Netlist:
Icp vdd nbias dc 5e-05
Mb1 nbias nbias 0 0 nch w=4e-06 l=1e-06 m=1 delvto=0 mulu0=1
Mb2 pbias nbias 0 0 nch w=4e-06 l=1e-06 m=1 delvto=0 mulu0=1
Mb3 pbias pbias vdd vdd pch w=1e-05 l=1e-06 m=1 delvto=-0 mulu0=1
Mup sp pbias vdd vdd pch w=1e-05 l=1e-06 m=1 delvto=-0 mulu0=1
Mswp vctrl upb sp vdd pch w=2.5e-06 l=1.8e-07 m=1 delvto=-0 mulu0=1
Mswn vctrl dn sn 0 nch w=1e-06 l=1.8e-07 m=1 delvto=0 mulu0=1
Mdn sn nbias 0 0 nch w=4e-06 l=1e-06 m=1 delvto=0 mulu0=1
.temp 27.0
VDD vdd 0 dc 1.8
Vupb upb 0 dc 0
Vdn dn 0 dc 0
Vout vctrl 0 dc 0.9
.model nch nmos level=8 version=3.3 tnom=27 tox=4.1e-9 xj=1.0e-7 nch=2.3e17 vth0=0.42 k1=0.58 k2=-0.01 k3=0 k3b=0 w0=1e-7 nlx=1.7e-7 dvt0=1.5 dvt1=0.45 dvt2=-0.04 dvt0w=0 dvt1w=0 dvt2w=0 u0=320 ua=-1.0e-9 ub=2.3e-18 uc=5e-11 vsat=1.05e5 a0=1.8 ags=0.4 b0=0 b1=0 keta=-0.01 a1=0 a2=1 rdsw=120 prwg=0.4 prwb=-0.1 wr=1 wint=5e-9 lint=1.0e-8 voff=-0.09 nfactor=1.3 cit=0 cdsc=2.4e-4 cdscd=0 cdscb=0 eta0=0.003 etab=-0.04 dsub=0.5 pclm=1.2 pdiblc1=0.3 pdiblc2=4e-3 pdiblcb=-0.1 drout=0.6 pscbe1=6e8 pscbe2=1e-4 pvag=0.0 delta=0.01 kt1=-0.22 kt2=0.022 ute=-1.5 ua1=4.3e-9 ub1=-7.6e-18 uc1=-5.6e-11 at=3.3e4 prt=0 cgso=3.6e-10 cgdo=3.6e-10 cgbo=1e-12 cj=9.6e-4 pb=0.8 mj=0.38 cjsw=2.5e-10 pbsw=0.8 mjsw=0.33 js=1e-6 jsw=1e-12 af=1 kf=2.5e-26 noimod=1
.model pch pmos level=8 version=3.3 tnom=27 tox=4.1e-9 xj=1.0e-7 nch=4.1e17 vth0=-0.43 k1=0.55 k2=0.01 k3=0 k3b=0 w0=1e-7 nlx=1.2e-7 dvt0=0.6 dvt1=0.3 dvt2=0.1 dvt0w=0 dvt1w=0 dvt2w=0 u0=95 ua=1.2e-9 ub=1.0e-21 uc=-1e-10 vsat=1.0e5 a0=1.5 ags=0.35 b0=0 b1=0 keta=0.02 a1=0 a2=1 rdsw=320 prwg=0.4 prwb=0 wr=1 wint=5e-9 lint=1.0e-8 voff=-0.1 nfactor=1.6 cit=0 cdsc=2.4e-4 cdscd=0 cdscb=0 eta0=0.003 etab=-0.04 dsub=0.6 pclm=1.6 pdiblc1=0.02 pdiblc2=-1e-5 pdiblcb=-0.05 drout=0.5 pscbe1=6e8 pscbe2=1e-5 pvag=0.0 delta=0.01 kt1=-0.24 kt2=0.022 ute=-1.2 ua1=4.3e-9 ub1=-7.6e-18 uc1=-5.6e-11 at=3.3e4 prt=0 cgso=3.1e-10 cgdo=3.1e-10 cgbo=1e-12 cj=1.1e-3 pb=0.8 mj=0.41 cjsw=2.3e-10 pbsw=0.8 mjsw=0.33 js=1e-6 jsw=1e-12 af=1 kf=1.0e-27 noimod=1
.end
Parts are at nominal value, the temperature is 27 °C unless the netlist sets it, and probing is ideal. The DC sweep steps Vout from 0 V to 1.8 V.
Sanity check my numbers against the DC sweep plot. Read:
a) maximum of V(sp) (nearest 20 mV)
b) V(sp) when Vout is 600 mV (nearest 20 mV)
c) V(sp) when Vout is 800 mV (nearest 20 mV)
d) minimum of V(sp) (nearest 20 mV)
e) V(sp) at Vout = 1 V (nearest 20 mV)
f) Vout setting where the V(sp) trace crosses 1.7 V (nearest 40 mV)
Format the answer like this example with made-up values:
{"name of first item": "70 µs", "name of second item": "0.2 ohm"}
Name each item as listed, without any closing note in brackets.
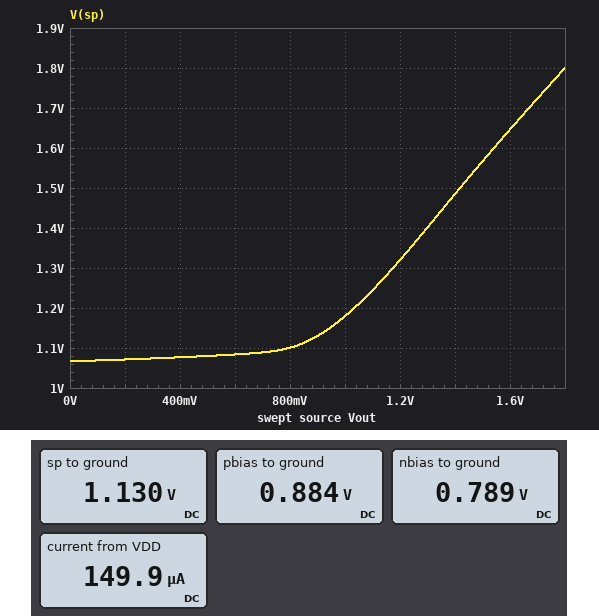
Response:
{"maximum of V(sp)": "1.80 V", "V(sp) when Vout is 600 mV": "1.08 V", "V(sp) when Vout is 800 mV": "1.10 V", "minimum of V(sp)": "1.06 V", "V(sp) at Vout = 1 V": "1.18 V", "Vout setting where the V(sp) trace crosses 1.7 V": "1.68 V"}
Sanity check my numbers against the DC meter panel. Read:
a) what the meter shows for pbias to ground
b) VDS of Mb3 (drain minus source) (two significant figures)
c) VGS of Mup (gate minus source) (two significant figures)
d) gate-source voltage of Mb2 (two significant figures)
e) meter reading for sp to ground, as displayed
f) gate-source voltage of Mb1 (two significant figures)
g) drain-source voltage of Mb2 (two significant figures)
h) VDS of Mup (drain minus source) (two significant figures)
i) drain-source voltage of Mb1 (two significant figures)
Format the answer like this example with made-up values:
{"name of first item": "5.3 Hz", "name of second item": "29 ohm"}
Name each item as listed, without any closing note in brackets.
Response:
{"what the meter shows for pbias to ground": "0.884 V", "VDS of Mb3 (drain minus source)": "-920 mV", "VGS of Mup (gate minus source)": "-920 mV", "gate-source voltage of Mb2": "790 mV", "meter reading for sp to ground, as displayed": "1.130 V", "gate-source voltage of Mb1": "790 mV", "drain-source voltage of Mb2": "880 mV", "VDS of Mup (drain minus source)": "-670 mV", "drain-source voltage of Mb1": "790 mV"}
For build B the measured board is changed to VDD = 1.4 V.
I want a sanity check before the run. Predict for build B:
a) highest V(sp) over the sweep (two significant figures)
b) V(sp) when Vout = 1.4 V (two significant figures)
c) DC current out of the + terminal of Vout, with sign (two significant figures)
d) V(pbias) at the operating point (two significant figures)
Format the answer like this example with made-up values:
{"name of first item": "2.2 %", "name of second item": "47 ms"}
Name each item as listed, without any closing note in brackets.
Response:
{"highest V(sp) over the sweep": "1.7 V", "V(sp) when Vout = 1.4 V": "1.4 V", "DC current out of the + terminal of Vout, with sign": "-46 µA", "V(pbias) at the operating point": "490 mV"}
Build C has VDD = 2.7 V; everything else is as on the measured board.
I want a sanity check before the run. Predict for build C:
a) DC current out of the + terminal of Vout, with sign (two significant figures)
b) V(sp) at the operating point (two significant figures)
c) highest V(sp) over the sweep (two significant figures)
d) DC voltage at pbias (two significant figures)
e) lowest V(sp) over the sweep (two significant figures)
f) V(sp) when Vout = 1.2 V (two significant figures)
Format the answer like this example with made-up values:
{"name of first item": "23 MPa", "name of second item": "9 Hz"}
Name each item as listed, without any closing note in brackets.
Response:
{"DC current out of the + terminal of Vout, with sign": "-52 µA", "V(sp) at the operating point": "1.3 V", "highest V(sp) over the sweep": "1.9 V", "DC voltage at pbias": "1.8 V", "lowest V(sp) over the sweep": "1.2 V", "V(sp) when Vout = 1.2 V": "1.4 V"}
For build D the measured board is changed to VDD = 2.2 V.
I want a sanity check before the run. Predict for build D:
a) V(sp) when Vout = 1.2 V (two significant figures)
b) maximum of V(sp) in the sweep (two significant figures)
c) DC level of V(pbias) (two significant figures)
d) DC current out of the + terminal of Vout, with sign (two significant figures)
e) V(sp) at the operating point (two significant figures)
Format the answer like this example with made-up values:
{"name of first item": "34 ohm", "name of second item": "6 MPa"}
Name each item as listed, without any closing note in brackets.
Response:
{"V(sp) when Vout = 1.2 V": "1.3 V", "maximum of V(sp) in the sweep": "1.9 V", "DC level of V(pbias)": "1.3 V", "DC current out of the + terminal of Vout, with sign": "-51 µA", "V(sp) at the operating point": "1.2 V"}
